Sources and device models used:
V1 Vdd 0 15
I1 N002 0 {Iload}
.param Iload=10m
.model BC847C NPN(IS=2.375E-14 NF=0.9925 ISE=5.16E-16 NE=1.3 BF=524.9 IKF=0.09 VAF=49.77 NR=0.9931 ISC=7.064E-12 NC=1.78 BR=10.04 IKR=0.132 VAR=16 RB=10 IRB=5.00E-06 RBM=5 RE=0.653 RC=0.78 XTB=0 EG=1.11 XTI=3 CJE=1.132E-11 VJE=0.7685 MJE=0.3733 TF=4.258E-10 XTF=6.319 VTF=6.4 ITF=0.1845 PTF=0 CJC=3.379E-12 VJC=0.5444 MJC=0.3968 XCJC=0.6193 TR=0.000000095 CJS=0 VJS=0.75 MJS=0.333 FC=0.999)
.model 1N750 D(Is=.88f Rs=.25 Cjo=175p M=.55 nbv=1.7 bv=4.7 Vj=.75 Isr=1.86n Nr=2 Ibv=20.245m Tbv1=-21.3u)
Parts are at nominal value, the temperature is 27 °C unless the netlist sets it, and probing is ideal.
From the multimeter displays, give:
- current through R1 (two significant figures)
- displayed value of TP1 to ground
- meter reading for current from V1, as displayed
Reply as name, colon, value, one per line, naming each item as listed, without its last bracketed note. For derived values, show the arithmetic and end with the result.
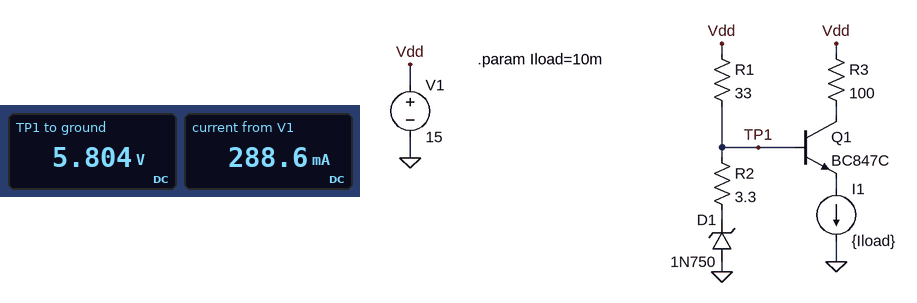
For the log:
current through R1: (15 V - 5.804 V) / 33 Ω = 280 mA
displayed value of TP1 to ground: 5.804 V
meter reading for current from V1, as displayed: 288.6 mA
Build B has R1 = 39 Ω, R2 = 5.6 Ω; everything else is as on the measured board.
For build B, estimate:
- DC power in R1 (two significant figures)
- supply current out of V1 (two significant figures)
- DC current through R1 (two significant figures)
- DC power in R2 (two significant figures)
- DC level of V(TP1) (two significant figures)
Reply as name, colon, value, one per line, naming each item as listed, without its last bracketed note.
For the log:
DC power in R1: 2.0 W
supply current out of V1: 240 mA
DC current through R1: 230 mA
DC power in R2: 290 mW
DC level of V(TP1): 6.1 V
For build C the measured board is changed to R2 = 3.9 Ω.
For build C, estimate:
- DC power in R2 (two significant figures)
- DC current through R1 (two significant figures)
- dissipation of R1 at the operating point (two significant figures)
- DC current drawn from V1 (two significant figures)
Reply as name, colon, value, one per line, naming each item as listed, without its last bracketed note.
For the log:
DC power in R2: 290 mW
DC current through R1: 270 mA
dissipation of R1 at the operating point: 2.5 W
DC current drawn from V1: 280 mA
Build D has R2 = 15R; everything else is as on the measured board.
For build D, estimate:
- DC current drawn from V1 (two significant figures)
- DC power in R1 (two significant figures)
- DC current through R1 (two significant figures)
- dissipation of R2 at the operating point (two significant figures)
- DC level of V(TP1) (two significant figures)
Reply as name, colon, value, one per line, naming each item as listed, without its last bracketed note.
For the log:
DC current drawn from V1: 220 mA
DC power in R1: 1.5 W
DC current through R1: 210 mA
dissipation of R2 at the operating point: 670 mW
DC level of V(TP1): 8.0 V
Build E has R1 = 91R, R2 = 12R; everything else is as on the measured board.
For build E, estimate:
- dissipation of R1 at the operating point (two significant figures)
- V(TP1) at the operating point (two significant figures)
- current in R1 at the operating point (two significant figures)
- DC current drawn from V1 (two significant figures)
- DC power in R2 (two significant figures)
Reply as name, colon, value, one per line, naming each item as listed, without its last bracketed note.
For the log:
dissipation of R1 at the operating point: 890 mW
V(TP1) at the operating point: 6.0 V
current in R1 at the operating point: 99 mA
DC current drawn from V1: 110 mA
DC power in R2: 120 mW
